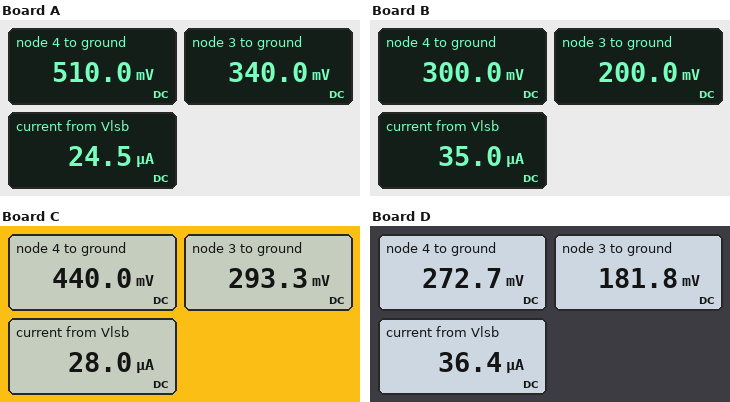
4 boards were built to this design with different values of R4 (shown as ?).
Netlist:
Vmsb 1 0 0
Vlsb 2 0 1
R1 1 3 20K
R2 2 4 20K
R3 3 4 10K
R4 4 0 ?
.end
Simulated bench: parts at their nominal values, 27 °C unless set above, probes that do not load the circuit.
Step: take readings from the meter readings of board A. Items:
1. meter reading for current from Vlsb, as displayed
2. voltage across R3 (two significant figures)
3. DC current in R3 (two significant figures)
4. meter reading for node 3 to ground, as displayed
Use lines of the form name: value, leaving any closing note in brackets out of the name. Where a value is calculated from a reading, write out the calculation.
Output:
meter reading for current from Vlsb, as displayed: 24.5 µA
voltage across R3: 510 mV - 340 mV = 170 mV
DC current in R3: (510 mV - 340 mV) / 10 kΩ = 17 µA
meter reading for node 3 to ground, as displayed: 340.0 mV
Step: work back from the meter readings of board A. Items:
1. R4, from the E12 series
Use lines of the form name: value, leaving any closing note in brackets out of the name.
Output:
R4, from the E12 series: 68 kΩ
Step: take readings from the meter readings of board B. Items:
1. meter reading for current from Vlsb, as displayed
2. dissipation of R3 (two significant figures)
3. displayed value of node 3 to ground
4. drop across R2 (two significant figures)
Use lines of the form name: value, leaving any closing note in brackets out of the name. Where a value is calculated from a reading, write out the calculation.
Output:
meter reading for current from Vlsb, as displayed: 35.0 µA
dissipation of R3: (300 mV - 200 mV)^2 / 10 kΩ = 1.0 µW
displayed value of node 3 to ground: 200.0 mV
drop across R2: 1 V - 300 mV = 700 mV
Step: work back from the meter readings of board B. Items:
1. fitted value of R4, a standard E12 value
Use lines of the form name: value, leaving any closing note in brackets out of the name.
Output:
fitted value of R4, a standard E12 value: 12 kΩ
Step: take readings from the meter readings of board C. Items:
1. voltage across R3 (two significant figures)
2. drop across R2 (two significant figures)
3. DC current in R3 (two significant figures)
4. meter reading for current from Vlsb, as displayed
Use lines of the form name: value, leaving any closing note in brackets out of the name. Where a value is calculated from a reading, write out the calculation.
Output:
voltage across R3: 440 mV - 293.3 mV = 150 mV
drop across R2: 1 V - 440 mV = 560 mV
DC current in R3: (440 mV - 293.3 mV) / 10 kΩ = 15 µA
meter reading for current from Vlsb, as displayed: 28.0 µA
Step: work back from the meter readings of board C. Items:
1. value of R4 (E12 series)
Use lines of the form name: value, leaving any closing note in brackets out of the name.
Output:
value of R4: 33 kΩ
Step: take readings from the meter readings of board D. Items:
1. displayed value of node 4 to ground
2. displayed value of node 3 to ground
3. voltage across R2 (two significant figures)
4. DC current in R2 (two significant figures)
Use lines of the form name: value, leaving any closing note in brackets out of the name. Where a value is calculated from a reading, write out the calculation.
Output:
displayed value of node 4 to ground: 272.7 mV
displayed value of node 3 to ground: 181.8 mV
voltage across R2: 1 V - 272.7 mV = 730 mV
DC current in R2: (1 V - 272.7 mV) / 20 kΩ = 36 µA
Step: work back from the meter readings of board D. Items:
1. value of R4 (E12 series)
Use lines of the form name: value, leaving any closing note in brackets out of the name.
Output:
value of R4: 10 kΩ
